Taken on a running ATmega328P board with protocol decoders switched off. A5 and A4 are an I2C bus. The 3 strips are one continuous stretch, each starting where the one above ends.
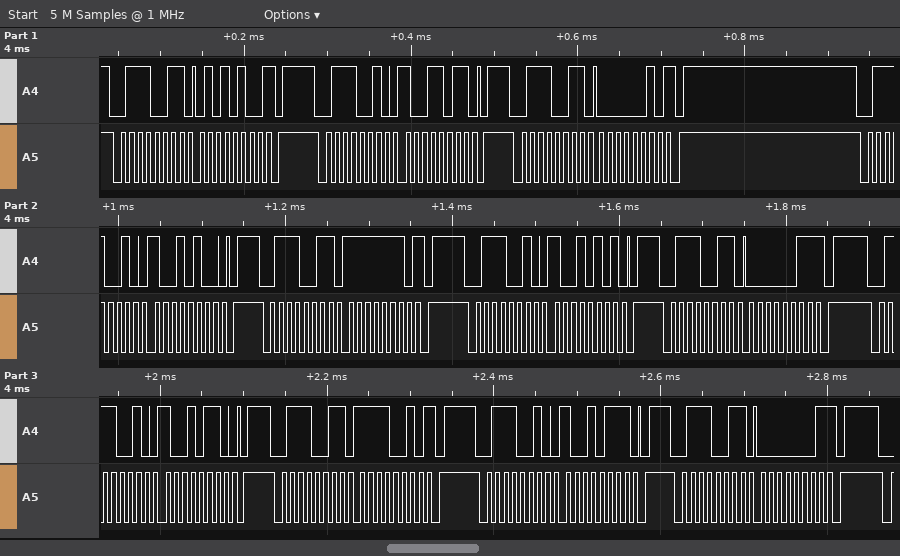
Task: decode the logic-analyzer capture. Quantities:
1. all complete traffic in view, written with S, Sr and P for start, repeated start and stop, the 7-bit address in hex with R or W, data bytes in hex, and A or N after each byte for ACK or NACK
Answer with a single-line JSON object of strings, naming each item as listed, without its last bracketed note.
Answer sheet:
{"all complete traffic in view, written with S, Sr and P for start, repeated start and stop, the 7-bit address in hex with R or W, data bytes in hex, and A or N after each byte for ACK or NACK": "S 39R A 54 N P S 39W A 9B A P S 39R A 02 N P S 39W A 94 A P S 39R A FE N P S 39W A 95 A P S 39R A 03 N P S 39W A 96 A P S 39R A F2 N P S 39W A 97 A P S 39R A 01 N P"}
